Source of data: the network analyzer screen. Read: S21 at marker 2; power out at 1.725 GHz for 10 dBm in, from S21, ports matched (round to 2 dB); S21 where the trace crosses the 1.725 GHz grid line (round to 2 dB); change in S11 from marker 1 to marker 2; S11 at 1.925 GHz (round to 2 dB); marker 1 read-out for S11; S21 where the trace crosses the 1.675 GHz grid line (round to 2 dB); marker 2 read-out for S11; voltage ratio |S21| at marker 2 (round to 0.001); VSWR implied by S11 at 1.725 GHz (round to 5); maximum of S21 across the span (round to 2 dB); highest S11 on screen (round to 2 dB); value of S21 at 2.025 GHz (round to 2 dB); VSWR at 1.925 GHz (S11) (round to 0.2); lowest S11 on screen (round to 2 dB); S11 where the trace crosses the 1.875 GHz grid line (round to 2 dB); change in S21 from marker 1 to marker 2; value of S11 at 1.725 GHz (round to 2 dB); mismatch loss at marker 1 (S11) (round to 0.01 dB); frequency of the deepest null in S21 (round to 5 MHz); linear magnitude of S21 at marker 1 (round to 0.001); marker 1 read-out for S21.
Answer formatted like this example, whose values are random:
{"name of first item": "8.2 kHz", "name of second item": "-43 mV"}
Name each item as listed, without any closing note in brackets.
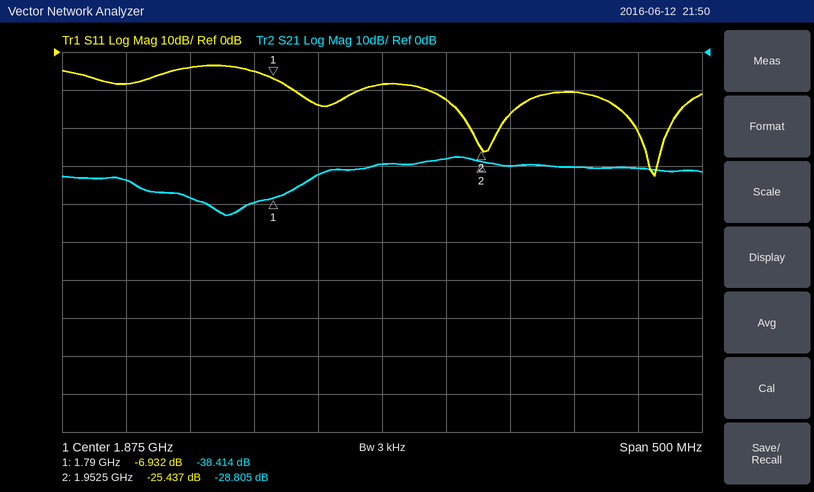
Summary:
{"S21 at marker 2": "-28.805 dB", "power out at 1.725 GHz for 10 dBm in, from S21, ports matched": "-28 dBm", "S21 where the trace crosses the 1.725 GHz grid line": "-38 dB", "change in S11 from marker 1 to marker 2": "-18.505 dB", "S11 at 1.925 GHz": "-12 dB", "marker 1 read-out for S11": "-6.932 dB", "S21 where the trace crosses the 1.675 GHz grid line": "-34 dB", "marker 2 read-out for S11": "-25.437 dB", "voltage ratio |S21| at marker 2": "0.036", "VSWR implied by S11 at 1.725 GHz": "5", "maximum of S21 across the span": "-28 dB", "highest S11 on screen": "-4 dB", "value of S21 at 2.025 GHz": "-30 dB", "VSWR at 1.925 GHz (S11)": "1.6", "lowest S11 on screen": "-32 dB", "S11 where the trace crosses the 1.875 GHz grid line": "-8 dB", "change in S21 from marker 1 to marker 2": "9.609 dB", "value of S11 at 1.725 GHz": "-4 dB", "mismatch loss at marker 1 (S11)": "0.98 dB", "frequency of the deepest null in S21": "1.755 GHz", "linear magnitude of S21 at marker 1": "0.012", "marker 1 read-out for S21": "-38.414 dB"}
